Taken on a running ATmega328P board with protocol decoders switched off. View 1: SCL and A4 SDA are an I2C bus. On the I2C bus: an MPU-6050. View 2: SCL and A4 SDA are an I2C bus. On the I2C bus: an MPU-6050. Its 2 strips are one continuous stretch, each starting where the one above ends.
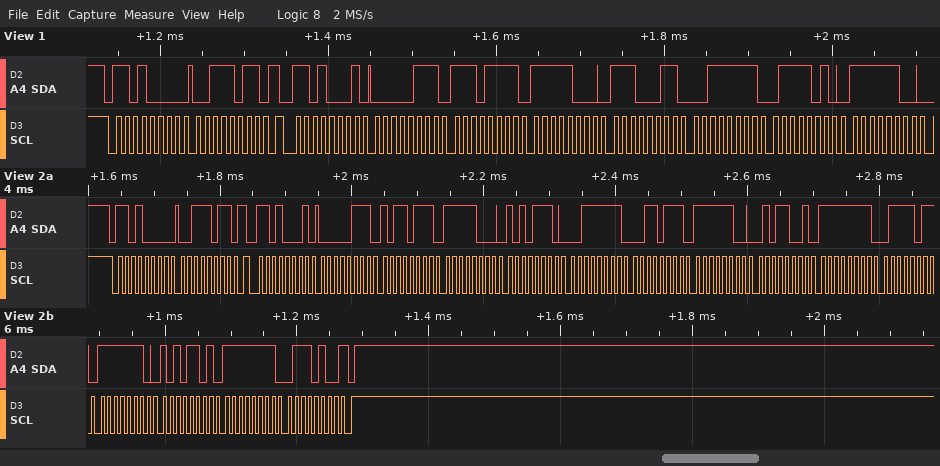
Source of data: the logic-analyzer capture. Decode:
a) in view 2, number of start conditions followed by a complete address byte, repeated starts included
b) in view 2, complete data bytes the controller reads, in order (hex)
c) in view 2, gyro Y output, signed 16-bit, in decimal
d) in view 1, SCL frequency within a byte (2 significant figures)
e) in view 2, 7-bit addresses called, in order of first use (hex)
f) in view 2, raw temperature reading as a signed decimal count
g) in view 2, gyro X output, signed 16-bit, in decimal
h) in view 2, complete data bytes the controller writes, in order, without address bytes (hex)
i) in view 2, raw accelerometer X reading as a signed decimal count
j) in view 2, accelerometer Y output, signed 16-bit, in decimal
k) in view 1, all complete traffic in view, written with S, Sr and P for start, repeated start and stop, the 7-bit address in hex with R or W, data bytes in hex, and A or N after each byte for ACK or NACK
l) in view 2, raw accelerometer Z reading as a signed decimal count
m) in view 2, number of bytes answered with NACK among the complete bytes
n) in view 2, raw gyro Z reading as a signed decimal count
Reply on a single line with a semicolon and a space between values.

2; 07 B7 F8 AE 3F 37 FC 59 FF 7B FE AD FF 74; -339; 100 kHz; 0x68; -935; -133; 3B; 1975; -1874; S 68W A 3B A Sr 68R A 07 A EF A F8 A E3 A 3F A 7A A FC A; 16183; 1; -140
